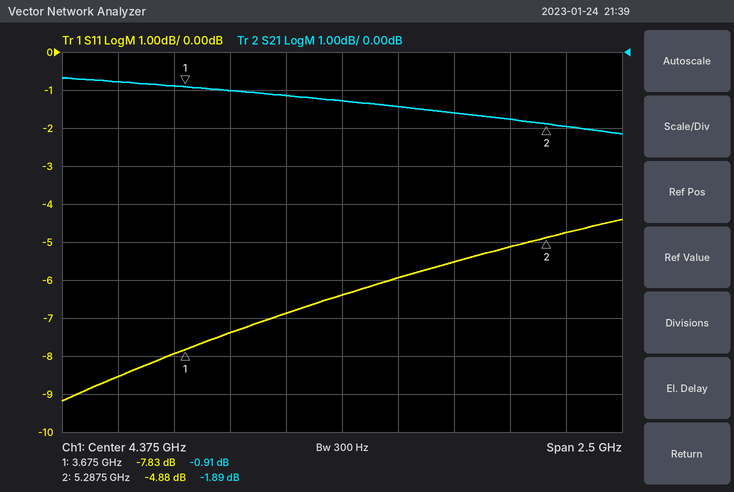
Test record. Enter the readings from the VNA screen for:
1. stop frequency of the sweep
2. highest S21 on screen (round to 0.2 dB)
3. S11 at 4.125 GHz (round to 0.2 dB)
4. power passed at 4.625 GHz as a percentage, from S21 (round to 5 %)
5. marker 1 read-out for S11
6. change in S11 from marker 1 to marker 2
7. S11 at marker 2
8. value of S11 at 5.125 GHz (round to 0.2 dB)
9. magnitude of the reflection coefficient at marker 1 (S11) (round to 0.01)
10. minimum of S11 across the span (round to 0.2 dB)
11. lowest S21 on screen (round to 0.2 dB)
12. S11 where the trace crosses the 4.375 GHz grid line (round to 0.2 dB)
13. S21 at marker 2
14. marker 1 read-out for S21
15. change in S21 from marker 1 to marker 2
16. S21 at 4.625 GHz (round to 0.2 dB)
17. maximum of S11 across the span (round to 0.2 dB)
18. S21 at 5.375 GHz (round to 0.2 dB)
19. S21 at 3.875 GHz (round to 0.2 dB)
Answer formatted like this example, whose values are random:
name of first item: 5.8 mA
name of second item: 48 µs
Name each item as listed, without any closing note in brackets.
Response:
stop frequency of the sweep: 5.625 GHz
highest S21 on screen: -0.6 dB
S11 at 4.125 GHz: -6.8 dB
power passed at 4.625 GHz as a percentage, from S21: 70 %
marker 1 read-out for S11: -7.83 dB
change in S11 from marker 1 to marker 2: 2.95 dB
S11 at marker 2: -4.88 dB
value of S11 at 5.125 GHz: -5.2 dB
magnitude of the reflection coefficient at marker 1 (S11): 0.41
minimum of S11 across the span: -9.2 dB
lowest S21 on screen: -2.2 dB
S11 where the trace crosses the 4.375 GHz grid line: -6.4 dB
S21 at marker 2: -1.89 dB
marker 1 read-out for S21: -0.91 dB
change in S21 from marker 1 to marker 2: -0.98 dB
S21 at 4.625 GHz: -1.4 dB
maximum of S11 across the span: -4.4 dB
S21 at 5.375 GHz: -2.0 dB
S21 at 3.875 GHz: -1.0 dB
